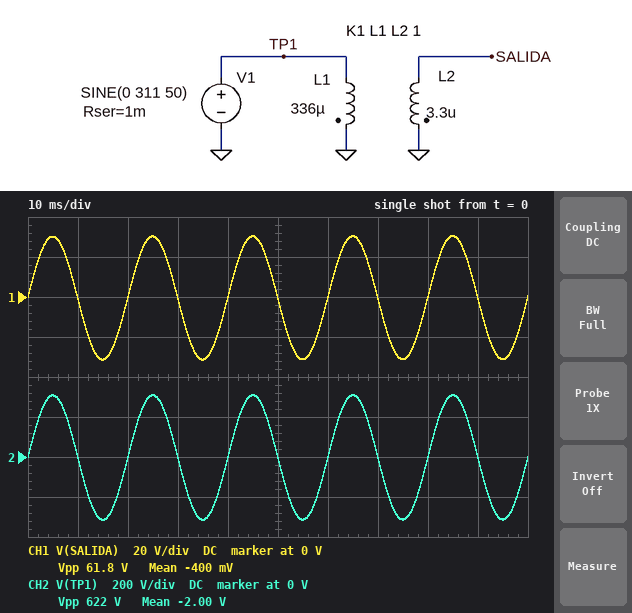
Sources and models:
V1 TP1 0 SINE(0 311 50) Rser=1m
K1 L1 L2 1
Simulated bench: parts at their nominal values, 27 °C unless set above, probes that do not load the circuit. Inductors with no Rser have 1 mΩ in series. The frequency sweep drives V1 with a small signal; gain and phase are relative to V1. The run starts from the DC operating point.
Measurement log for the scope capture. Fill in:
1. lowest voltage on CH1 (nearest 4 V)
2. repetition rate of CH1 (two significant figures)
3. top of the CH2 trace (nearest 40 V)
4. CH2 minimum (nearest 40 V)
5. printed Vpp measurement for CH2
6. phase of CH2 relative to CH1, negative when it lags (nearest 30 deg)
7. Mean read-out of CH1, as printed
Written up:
-32 V
50 Hz
320 V
-320 V
622 V
0 deg
-400 mV
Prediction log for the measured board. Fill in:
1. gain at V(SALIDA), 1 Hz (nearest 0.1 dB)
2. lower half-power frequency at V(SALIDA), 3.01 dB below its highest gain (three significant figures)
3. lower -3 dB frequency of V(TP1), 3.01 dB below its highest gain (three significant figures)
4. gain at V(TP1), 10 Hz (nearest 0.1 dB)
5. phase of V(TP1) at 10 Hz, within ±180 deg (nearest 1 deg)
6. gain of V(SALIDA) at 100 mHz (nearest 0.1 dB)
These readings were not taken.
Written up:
-22.9 dB
947 mHz
670 mHz
0 dB
3 deg
-39.7 dB
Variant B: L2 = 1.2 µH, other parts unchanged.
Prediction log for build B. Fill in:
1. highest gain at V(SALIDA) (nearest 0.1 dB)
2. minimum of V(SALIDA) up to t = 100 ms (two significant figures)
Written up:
-24.5 dB
-19 V
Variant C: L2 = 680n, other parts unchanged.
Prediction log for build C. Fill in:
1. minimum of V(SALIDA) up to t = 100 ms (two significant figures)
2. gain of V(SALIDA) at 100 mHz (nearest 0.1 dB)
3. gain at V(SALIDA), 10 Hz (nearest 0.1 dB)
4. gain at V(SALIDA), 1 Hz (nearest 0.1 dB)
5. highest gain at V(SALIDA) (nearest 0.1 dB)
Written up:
-14 V
-46.5 dB
-27.0 dB
-29.7 dB
-26.9 dB
